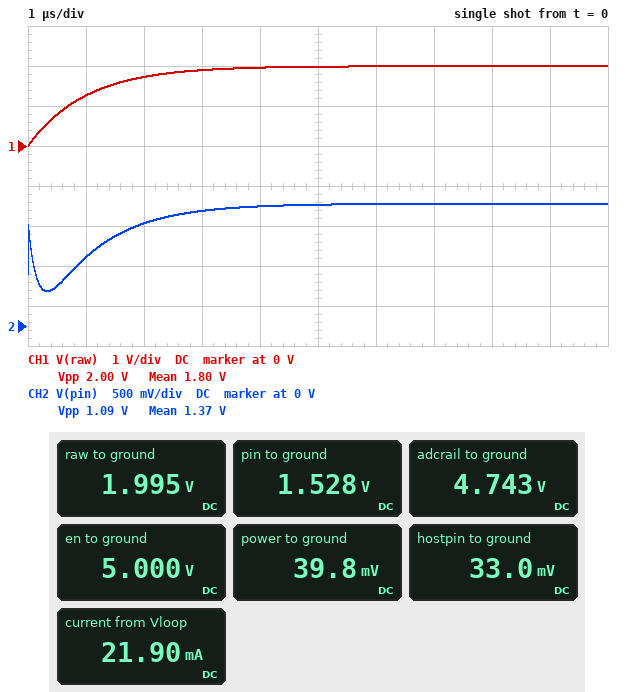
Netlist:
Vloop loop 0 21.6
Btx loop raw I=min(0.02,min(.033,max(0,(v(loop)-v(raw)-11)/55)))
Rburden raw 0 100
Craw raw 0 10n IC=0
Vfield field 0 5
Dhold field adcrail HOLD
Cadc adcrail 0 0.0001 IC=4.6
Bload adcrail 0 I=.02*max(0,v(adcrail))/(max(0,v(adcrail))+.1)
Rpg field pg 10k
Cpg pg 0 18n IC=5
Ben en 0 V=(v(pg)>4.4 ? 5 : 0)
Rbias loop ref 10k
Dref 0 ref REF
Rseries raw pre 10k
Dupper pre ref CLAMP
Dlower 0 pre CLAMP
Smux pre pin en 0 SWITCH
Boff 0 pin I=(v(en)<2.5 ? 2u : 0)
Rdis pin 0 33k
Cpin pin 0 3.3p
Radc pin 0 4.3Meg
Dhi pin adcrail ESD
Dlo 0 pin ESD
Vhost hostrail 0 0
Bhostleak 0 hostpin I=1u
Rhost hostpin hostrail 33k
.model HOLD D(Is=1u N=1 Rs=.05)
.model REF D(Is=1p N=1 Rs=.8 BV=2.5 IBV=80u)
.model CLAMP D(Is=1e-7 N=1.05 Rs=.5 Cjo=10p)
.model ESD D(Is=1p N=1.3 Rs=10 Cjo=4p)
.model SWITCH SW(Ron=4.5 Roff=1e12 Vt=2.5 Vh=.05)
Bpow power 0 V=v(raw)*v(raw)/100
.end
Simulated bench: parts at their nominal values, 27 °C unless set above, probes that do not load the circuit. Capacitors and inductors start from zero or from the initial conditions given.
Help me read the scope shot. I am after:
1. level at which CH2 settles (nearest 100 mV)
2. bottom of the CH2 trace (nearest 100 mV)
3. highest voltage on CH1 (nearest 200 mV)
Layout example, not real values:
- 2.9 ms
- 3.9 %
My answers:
- 1.5 V
- 400 mV
- 2.0 V
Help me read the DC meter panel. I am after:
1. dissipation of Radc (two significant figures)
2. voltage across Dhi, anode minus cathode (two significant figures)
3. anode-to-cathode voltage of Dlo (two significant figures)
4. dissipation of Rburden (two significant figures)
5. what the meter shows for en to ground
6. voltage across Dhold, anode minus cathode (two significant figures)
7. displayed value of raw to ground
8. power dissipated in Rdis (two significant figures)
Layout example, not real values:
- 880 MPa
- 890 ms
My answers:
- 540 nW
- -3.2 V
- -1.5 V
- 40 mW
- 5.000 V
- 260 mV
- 1.995 V
- 71 µW
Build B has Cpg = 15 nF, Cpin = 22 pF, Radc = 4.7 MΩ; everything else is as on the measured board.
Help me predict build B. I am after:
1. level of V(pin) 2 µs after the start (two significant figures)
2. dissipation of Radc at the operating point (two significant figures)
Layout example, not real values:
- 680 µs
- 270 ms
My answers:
- 1.2 V
- 500 nW
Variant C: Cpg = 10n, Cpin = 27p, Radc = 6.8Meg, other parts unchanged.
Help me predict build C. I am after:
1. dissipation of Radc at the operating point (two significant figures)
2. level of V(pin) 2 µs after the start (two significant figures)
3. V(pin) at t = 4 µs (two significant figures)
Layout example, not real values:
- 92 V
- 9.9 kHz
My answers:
- 340 nW
- 1.2 V
- 1.5 V
